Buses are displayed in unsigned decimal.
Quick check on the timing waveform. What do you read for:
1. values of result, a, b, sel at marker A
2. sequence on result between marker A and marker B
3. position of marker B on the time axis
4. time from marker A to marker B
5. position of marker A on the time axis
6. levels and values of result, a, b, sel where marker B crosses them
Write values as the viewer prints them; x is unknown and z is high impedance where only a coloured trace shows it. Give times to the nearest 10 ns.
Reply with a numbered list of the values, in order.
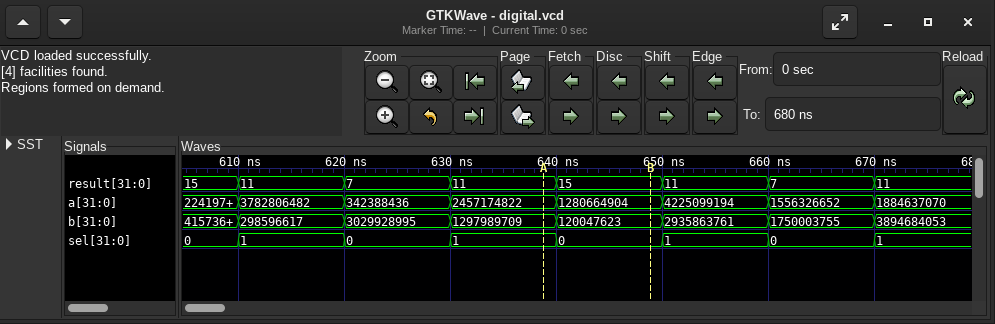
1. result=11, a=2457174822, b=1297989709, sel=1
2. 11, 15
3. 650 ns
4. 10 ns
5. 640 ns
6. result=15, a=1280664904, b=120047623, sel=0
